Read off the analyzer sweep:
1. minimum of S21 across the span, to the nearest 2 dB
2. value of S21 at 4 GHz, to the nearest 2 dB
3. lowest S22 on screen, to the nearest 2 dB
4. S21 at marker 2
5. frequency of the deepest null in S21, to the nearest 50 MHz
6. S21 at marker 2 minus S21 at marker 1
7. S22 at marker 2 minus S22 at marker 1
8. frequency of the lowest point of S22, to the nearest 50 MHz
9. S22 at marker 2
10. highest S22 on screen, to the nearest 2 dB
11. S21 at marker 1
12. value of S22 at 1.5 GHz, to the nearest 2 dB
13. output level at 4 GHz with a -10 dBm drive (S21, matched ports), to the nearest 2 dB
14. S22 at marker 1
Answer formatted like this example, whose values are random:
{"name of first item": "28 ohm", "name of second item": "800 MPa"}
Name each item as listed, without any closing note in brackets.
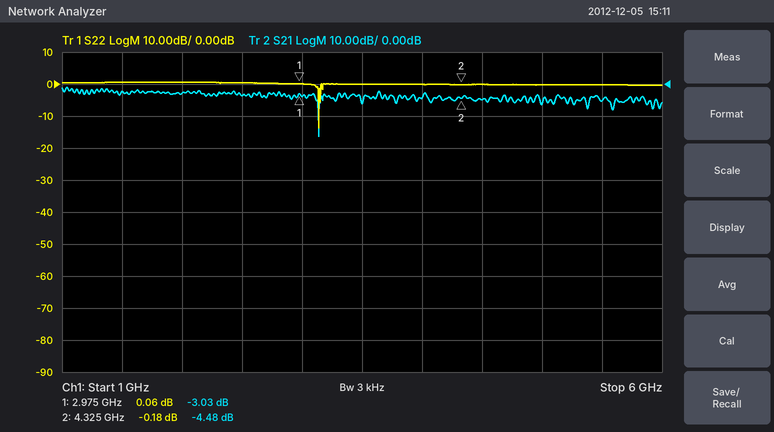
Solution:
{"minimum of S21 across the span, to the nearest 2 dB": "-16 dB", "value of S21 at 4 GHz, to the nearest 2 dB": "-4 dB", "lowest S22 on screen, to the nearest 2 dB": "-14 dB", "S21 at marker 2": "-4.48 dB", "frequency of the deepest null in S21, to the nearest 50 MHz": "3.15 GHz", "S21 at marker 2 minus S21 at marker 1": "-1.45 dB", "S22 at marker 2 minus S22 at marker 1": "-0.24 dB", "frequency of the lowest point of S22, to the nearest 50 MHz": "3.15 GHz", "S22 at marker 2": "-0.18 dB", "highest S22 on screen, to the nearest 2 dB": "0 dB", "S21 at marker 1": "-3.03 dB", "value of S22 at 1.5 GHz, to the nearest 2 dB": "0 dB", "output level at 4 GHz with a -10 dBm drive (S21, matched ports), to the nearest 2 dB": "-14 dBm", "S22 at marker 1": "0.06 dB"}
